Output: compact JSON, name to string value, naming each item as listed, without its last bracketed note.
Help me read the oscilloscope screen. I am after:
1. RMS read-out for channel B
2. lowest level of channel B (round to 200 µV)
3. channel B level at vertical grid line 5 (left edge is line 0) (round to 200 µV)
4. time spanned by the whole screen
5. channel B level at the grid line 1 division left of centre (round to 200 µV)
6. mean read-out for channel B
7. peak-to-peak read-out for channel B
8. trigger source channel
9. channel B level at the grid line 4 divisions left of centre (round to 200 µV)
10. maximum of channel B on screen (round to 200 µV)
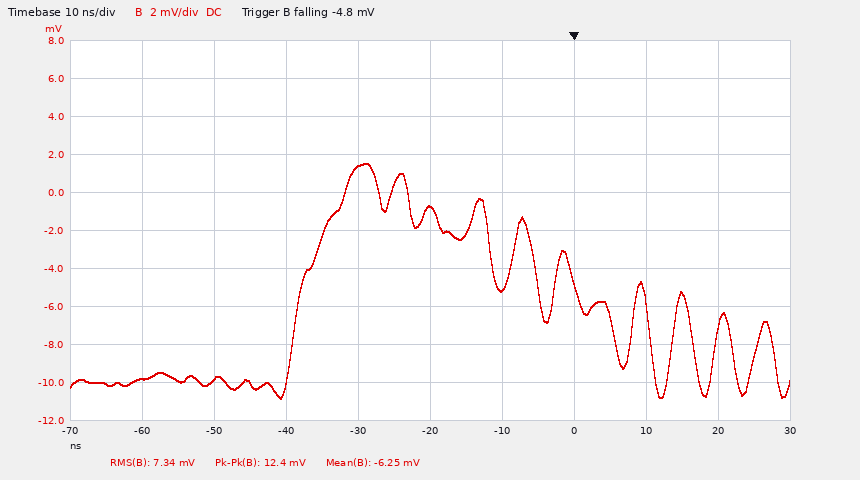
{"RMS read-out for channel B": "7.34 mV", "lowest level of channel B": "-10.8 mV", "channel B level at vertical grid line 5 (left edge is line 0)": "-800 µV", "time spanned by the whole screen": "100 ns", "channel B level at the grid line 1 division left of centre": "1.4 mV", "mean read-out for channel B": "-6.25 mV", "peak-to-peak read-out for channel B": "12.4 mV", "trigger source channel": "channel B", "channel B level at the grid line 4 divisions left of centre": "-9.8 mV", "maximum of channel B on screen": "1.6 mV"}
